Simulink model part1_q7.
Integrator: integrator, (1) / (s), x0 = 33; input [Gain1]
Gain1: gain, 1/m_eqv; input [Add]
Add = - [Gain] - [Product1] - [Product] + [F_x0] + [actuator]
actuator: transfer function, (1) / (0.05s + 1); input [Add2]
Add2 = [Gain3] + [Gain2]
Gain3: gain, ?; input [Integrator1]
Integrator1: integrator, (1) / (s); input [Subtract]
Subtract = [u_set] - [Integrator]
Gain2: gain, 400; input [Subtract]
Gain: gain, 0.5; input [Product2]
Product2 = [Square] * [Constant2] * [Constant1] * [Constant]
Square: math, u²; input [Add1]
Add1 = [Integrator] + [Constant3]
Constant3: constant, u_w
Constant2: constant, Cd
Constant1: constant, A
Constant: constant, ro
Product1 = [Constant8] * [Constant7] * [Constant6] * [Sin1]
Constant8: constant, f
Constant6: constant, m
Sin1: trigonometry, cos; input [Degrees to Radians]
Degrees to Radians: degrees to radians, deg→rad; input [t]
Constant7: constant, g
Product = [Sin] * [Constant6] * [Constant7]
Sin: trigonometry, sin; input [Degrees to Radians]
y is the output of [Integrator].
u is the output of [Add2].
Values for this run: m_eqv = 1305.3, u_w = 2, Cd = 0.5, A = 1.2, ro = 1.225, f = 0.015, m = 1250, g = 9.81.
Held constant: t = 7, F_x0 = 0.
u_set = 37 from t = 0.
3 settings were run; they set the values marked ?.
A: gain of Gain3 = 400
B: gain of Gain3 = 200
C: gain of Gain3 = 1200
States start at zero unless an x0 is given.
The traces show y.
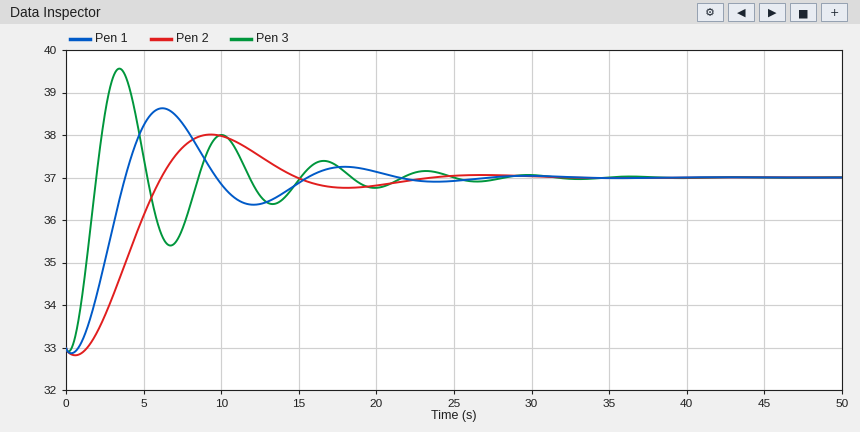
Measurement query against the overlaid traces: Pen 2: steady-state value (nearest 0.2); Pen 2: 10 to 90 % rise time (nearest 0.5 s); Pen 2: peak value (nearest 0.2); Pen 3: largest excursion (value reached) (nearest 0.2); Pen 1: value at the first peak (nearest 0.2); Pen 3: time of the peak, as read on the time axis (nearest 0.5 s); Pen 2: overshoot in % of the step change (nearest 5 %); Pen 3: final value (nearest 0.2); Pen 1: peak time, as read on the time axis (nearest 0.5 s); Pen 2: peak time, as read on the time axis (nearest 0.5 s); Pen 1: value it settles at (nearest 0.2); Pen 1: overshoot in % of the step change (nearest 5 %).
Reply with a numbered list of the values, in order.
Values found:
1. 37.0
2. 3.5 s
3. 38.0
4. 39.6
5. 38.6
6. 3.5 s
7. 25 %
8. 37.0
9. 6.0 s
10. 9.5 s
11. 37.0
12. 40 %
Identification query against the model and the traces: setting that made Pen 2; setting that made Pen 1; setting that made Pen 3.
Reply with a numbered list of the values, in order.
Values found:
1. B
2. A
3. C
